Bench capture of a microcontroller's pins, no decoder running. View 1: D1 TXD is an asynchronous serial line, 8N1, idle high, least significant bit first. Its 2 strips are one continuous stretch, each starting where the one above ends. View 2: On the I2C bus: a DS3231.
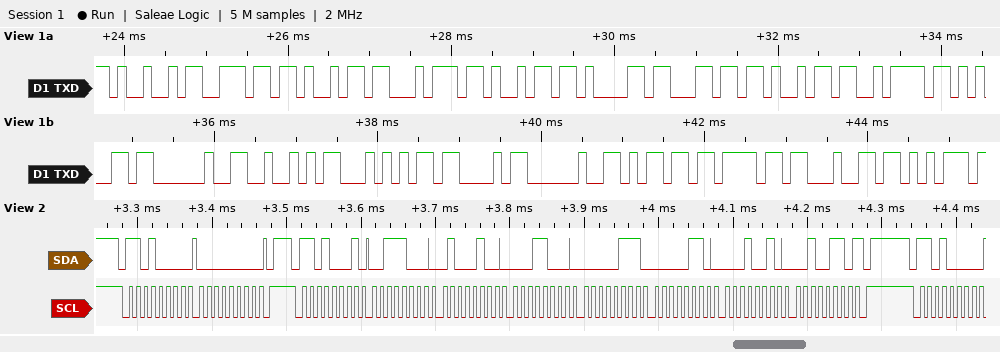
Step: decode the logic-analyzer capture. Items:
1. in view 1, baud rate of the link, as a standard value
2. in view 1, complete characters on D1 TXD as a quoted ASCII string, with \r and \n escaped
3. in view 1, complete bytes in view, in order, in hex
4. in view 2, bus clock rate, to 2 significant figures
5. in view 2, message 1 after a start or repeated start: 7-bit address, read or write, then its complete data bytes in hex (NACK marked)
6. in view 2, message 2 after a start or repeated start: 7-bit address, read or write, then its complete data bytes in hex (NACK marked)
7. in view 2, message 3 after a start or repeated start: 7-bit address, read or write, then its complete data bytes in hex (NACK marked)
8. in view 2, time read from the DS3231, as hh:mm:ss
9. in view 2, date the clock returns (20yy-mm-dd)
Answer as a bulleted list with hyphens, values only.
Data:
- 9600 baud
- "Initialize RTC modu"
- 49 6E 69 74 69 61 6C 69 7A 65 20 52 54 43 20 6D 6F 64 75
- 100 kHz
- 0x68 write: 00
- 0x68 read: 38 44 18 07 06 12 26 NACK
- 0x68 write
- 18:44:38
- 2026-12-06
